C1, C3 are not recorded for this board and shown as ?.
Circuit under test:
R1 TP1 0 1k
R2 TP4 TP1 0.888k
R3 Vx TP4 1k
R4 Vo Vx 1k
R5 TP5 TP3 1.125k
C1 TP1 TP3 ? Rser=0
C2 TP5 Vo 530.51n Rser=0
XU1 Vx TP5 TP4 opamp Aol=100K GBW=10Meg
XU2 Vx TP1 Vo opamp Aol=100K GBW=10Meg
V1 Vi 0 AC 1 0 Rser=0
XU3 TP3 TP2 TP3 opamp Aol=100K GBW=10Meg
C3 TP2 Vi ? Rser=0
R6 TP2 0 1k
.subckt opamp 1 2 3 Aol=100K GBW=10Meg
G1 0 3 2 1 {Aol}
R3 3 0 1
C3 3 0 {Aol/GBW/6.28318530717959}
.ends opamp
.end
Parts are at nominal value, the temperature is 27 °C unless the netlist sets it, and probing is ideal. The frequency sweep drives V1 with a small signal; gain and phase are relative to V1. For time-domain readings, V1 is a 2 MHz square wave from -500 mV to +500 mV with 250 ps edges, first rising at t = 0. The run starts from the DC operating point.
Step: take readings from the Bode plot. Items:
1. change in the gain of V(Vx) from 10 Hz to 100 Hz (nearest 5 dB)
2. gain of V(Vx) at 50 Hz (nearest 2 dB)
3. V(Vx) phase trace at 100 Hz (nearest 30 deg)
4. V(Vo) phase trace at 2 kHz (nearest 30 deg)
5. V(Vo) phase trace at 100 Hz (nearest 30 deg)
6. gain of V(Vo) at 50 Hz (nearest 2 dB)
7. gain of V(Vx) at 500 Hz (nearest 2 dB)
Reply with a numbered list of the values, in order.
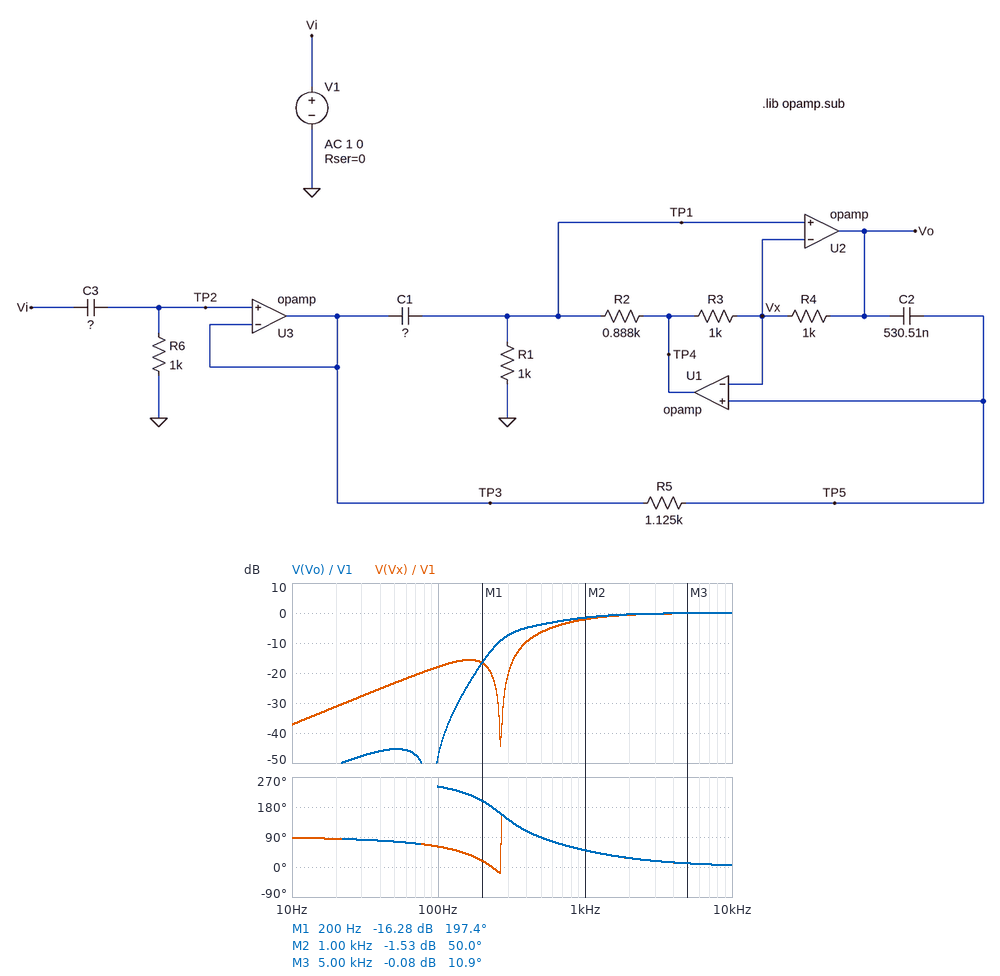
1. 20 dB
2. -24 dB
3. 60 deg
4. 30 deg
5. 240 deg
6. -46 dB
7. -6 dB
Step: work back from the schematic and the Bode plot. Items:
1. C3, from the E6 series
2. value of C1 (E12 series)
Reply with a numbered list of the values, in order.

1. 220 nF
2. 680 nF
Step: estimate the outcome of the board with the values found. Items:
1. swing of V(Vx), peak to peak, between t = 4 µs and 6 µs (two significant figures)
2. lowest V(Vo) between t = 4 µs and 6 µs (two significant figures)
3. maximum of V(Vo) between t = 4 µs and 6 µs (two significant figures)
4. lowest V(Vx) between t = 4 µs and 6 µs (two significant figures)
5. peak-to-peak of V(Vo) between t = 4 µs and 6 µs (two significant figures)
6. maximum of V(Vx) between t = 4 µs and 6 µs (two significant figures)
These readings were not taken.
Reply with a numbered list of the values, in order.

1. 1.1 V
2. -160 mV
3. 1.1 V
4. -61 mV
5. 1.3 V
6. 1.0 V
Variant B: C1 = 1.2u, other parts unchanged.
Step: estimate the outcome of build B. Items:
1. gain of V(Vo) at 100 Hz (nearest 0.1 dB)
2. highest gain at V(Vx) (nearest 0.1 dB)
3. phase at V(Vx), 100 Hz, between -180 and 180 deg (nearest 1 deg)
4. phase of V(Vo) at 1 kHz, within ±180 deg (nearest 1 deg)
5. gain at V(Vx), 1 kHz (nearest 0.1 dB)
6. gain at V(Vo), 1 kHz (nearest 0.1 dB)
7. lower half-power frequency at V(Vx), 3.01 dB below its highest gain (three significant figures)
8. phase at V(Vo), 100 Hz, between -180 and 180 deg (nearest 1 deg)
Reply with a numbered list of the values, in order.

1. -32.7 dB
2. 0 dB
3. 58 deg
4. 44 deg
5. -1.9 dB
6. -1.6 dB
7. 750 Hz
8. -122 deg
